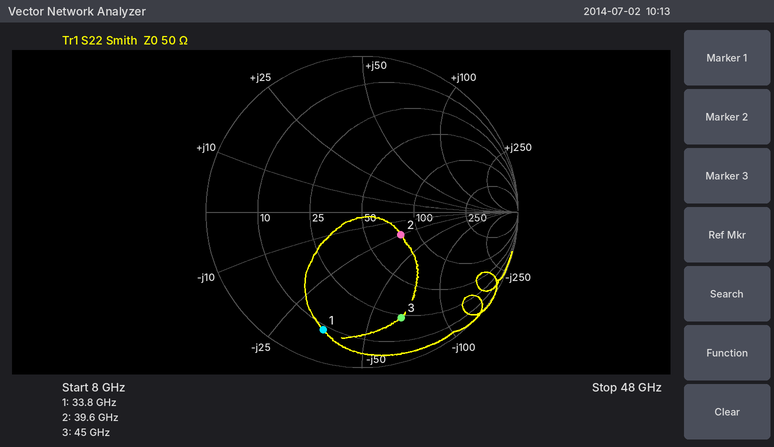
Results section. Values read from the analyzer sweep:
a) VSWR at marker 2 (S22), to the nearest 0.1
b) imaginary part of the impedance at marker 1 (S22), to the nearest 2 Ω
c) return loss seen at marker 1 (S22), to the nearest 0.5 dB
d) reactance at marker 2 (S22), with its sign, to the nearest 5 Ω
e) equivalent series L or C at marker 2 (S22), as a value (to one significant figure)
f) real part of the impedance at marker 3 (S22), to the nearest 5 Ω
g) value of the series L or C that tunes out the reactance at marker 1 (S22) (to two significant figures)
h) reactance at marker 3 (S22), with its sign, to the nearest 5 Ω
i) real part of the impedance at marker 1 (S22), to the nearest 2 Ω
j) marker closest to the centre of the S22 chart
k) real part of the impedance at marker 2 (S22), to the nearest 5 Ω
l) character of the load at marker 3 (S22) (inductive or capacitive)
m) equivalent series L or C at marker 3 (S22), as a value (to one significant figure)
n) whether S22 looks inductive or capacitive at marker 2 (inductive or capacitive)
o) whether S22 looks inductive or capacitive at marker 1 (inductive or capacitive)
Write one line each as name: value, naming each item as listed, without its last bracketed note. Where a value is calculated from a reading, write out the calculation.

VSWR at marker 2 (S22), to the nearest 0.1: 1.8
imaginary part of the impedance at marker 1 (S22), to the nearest 2 Ω: -36 Ω
return loss seen at marker 1 (S22), to the nearest 0.5 dB: 2.0 dB
reactance at marker 2 (S22), with its sign, to the nearest 5 Ω: -25 Ω
equivalent series L or C at marker 2 (S22), as a value: C = 1/(2π × 39.6 GHz × 25 Ω) ≈ 161 fF, so 200 fF to one significant figure
real part of the impedance at marker 3 (S22), to the nearest 5 Ω: 25 Ω
value of the series L or C that tunes out the reactance at marker 1 (S22): L = 36 Ω/(2π × 33.8 GHz) ≈ 170 pH
reactance at marker 3 (S22), with its sign, to the nearest 5 Ω: -65 Ω
real part of the impedance at marker 1 (S22), to the nearest 2 Ω: 8 Ω
marker closest to the centre of the S22 chart: marker 2
real part of the impedance at marker 2 (S22), to the nearest 5 Ω: 80 Ω
character of the load at marker 3 (S22): capacitive
equivalent series L or C at marker 3 (S22), as a value: C = 1/(2π × 45 GHz × 65 Ω) ≈ 54.4 fF, so 50 fF to one significant figure
whether S22 looks inductive or capacitive at marker 2: capacitive
whether S22 looks inductive or capacitive at marker 1: capacitive
